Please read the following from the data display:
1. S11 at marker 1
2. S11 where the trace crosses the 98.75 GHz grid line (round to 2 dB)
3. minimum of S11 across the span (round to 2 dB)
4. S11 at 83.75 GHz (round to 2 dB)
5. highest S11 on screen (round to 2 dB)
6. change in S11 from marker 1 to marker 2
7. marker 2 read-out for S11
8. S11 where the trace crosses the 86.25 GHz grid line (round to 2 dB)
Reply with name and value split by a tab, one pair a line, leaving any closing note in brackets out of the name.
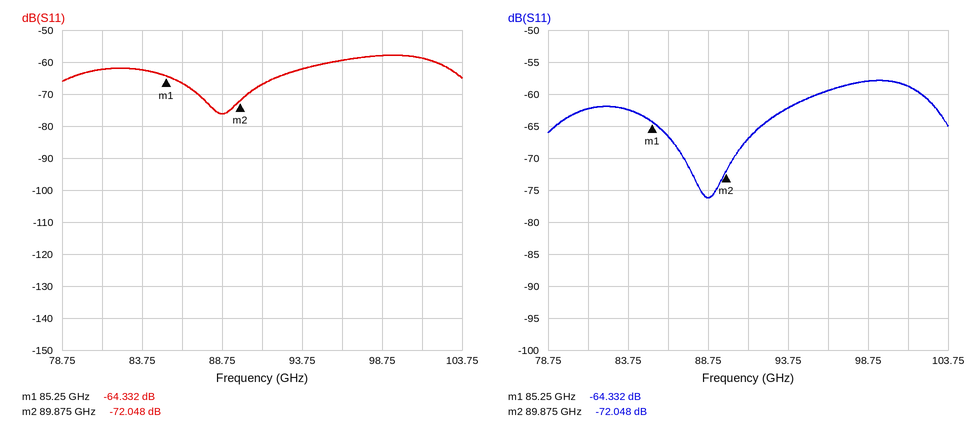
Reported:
S11 at marker 1	-64.332 dB
S11 where the trace crosses the 98.75 GHz grid line	-58 dB
minimum of S11 across the span	-76 dB
S11 at 83.75 GHz	-62 dB
highest S11 on screen	-58 dB
change in S11 from marker 1 to marker 2	-7.716 dB
marker 2 read-out for S11	-72.048 dB
S11 where the trace crosses the 86.25 GHz grid line	-66 dB
